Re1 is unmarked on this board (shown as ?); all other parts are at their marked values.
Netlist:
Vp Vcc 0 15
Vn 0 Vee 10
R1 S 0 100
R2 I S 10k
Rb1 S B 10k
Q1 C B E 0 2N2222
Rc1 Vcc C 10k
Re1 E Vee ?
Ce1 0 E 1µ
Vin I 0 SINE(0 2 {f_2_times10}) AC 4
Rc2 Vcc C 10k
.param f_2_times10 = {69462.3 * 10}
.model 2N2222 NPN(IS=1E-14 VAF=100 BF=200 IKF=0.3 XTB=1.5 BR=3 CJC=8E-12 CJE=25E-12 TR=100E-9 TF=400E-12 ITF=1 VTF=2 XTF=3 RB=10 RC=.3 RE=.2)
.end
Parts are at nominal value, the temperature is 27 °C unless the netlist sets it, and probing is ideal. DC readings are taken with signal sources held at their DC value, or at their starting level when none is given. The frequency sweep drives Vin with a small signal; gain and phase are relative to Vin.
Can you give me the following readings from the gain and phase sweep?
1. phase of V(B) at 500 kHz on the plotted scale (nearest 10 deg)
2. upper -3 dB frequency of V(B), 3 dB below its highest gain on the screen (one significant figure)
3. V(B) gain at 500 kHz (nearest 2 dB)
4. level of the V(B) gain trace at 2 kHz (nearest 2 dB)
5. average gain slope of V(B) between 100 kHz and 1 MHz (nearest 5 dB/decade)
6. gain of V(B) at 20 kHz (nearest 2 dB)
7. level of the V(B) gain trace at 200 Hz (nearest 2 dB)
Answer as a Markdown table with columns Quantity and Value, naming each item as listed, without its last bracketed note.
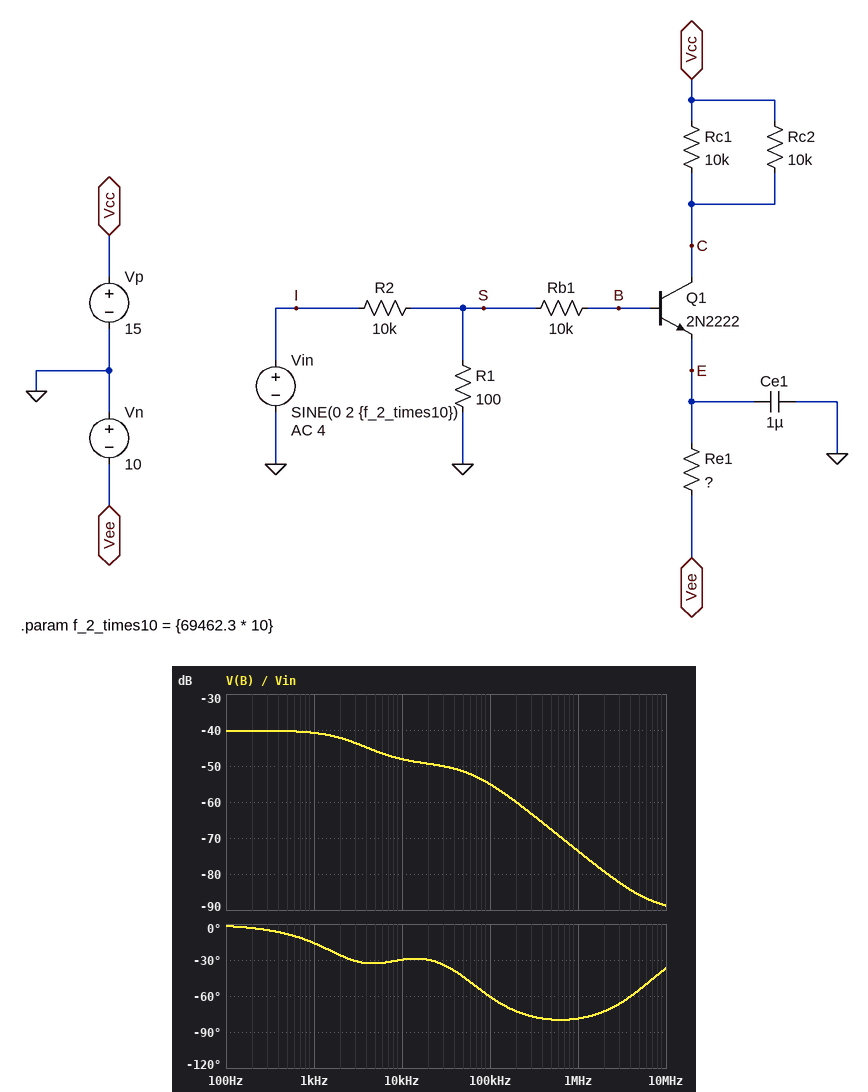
| Quantity | Value |
|---|---|
| phase of V(B) at 500 kHz on the plotted scale | -80 deg |
| upper -3 dB frequency of V(B), 3 dB below its highest gain on the screen | 3 kHz |
| V(B) gain at 500 kHz | -68 dB |
| level of the V(B) gain trace at 2 kHz | -42 dB |
| average gain slope of V(B) between 100 kHz and 1 MHz | -20 dB/decade |
| gain of V(B) at 20 kHz | -50 dB |
| level of the V(B) gain trace at 200 Hz | -40 dB |
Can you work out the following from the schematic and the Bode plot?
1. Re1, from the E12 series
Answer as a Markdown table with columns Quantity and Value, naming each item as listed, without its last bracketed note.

| Quantity | Value |
|---|---|
| Re1, from the E12 series | 8.2 kΩ |
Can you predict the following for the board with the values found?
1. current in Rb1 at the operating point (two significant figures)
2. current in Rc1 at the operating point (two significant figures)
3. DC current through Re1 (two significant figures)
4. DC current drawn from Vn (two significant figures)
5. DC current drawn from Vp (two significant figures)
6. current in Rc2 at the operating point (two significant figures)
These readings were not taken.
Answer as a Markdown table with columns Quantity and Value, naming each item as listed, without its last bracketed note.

| Quantity | Value |
|---|---|
| current in Rb1 at the operating point | 5.2 µA |
| current in Rc1 at the operating point | 560 µA |
| DC current through Re1 | 1.1 mA |
| DC current drawn from Vn | 1.1 mA |
| DC current drawn from Vp | 1.1 mA |
| current in Rc2 at the operating point | 560 µA |
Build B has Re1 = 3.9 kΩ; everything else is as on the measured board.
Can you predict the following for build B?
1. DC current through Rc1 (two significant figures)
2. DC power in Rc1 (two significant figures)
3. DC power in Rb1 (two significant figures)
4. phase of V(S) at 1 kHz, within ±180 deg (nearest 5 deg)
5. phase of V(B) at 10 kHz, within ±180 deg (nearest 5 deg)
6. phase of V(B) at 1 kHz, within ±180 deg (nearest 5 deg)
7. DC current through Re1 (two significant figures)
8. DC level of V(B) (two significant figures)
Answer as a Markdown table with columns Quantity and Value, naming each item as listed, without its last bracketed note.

| Quantity | Value |
|---|---|
| DC current through Rc1 | 1.2 mA |
| DC power in Rc1 | 14 mW |
| DC power in Rb1 | 1.3 µW |
| phase of V(S) at 1 kHz, within ±180 deg | 0 deg |
| phase of V(B) at 10 kHz, within ±180 deg | -50 deg |
| phase of V(B) at 1 kHz, within ±180 deg | -20 deg |
| DC current through Re1 | 2.4 mA |
| DC level of V(B) | -120 mV |
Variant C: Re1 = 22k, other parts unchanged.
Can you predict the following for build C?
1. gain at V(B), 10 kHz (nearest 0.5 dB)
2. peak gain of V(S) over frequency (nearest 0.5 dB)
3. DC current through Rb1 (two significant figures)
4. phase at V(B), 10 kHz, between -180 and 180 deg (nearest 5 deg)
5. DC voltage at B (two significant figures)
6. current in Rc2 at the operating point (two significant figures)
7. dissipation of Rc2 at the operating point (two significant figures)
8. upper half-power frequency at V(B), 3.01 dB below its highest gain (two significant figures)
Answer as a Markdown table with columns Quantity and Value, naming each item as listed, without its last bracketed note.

| Quantity | Value |
|---|---|
| gain at V(B), 10 kHz | -44.5 dB |
| peak gain of V(S) over frequency | -40.0 dB |
| DC current through Rb1 | 1.9 µA |
| phase at V(B), 10 kHz, between -180 and 180 deg | -10 deg |
| DC voltage at B | -19 mV |
| current in Rc2 at the operating point | 210 µA |
| dissipation of Rc2 at the operating point | 450 µW |
| upper half-power frequency at V(B), 3.01 dB below its highest gain | 2.7 kHz |
